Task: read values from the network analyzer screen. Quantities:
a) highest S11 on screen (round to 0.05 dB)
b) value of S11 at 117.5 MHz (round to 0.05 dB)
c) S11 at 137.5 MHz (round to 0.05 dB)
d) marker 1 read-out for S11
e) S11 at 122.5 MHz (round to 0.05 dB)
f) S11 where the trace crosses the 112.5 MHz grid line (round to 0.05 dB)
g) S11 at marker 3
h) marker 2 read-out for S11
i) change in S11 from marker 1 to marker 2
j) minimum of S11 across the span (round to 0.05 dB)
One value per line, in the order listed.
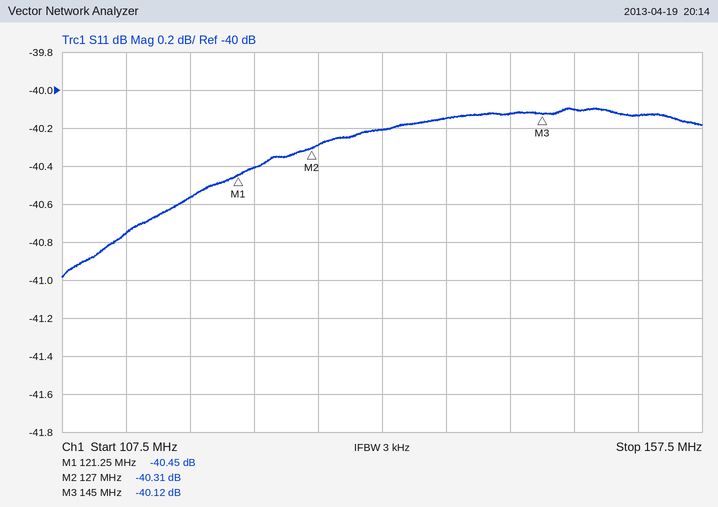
-40.10 dB
-40.55 dB
-40.15 dB
-40.45 dB
-40.40 dB
-40.75 dB
-40.12 dB
-40.31 dB
0.14 dB
-41.00 dB
